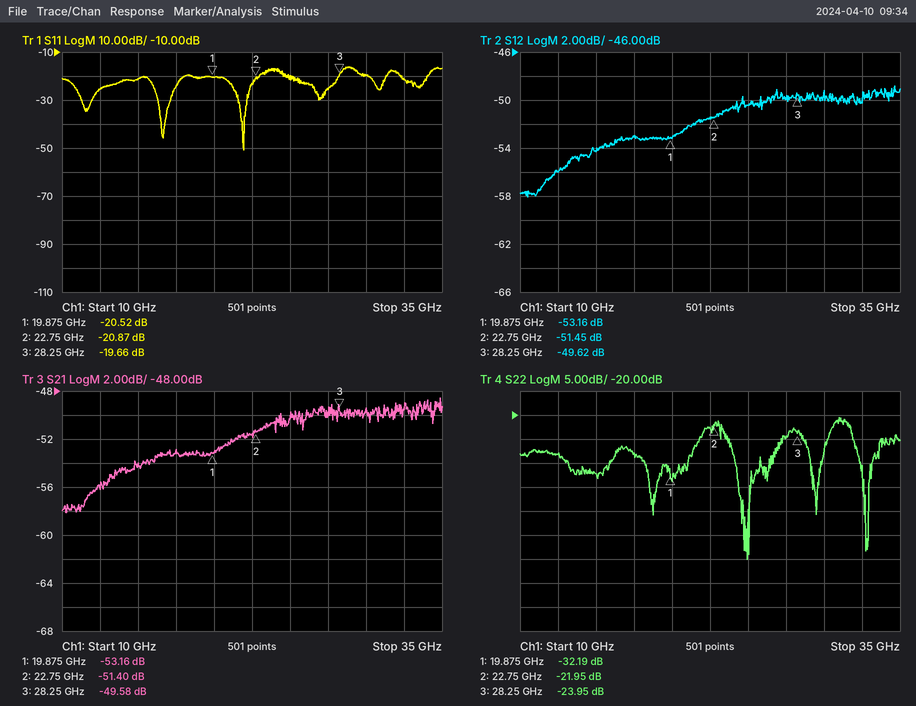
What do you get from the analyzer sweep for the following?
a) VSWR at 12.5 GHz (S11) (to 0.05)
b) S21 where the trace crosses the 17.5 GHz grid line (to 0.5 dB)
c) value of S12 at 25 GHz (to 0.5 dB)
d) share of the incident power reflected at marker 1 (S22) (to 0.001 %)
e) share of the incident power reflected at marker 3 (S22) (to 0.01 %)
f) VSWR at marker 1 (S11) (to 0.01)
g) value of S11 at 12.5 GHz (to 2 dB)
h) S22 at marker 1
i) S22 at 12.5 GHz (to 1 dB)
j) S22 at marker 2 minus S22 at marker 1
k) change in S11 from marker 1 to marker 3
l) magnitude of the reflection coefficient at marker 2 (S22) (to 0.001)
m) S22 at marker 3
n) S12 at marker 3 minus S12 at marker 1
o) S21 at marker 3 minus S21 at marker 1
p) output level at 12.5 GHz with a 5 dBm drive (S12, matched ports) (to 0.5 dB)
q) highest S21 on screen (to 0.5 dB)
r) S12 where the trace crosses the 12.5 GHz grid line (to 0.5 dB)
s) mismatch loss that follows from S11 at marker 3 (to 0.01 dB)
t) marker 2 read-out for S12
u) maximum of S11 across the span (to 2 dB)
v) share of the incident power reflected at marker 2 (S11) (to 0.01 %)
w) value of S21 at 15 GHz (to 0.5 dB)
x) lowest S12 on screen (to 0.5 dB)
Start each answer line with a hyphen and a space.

- 1.10
- -53.0 dB
- -50.5 dB
- 0.060 %
- 0.40 %
- 1.21
- -26 dB
- -32.19 dB
- -28 dB
- 10.24 dB
- 0.86 dB
- 0.080
- -23.95 dB
- 3.54 dB
- 3.58 dB
- -51.0 dBm
- -48.5 dB
- -56.0 dB
- 0.05 dB
- -51.45 dB
- -16 dB
- 0.82 %
- -54.0 dB
- -58.0 dB
